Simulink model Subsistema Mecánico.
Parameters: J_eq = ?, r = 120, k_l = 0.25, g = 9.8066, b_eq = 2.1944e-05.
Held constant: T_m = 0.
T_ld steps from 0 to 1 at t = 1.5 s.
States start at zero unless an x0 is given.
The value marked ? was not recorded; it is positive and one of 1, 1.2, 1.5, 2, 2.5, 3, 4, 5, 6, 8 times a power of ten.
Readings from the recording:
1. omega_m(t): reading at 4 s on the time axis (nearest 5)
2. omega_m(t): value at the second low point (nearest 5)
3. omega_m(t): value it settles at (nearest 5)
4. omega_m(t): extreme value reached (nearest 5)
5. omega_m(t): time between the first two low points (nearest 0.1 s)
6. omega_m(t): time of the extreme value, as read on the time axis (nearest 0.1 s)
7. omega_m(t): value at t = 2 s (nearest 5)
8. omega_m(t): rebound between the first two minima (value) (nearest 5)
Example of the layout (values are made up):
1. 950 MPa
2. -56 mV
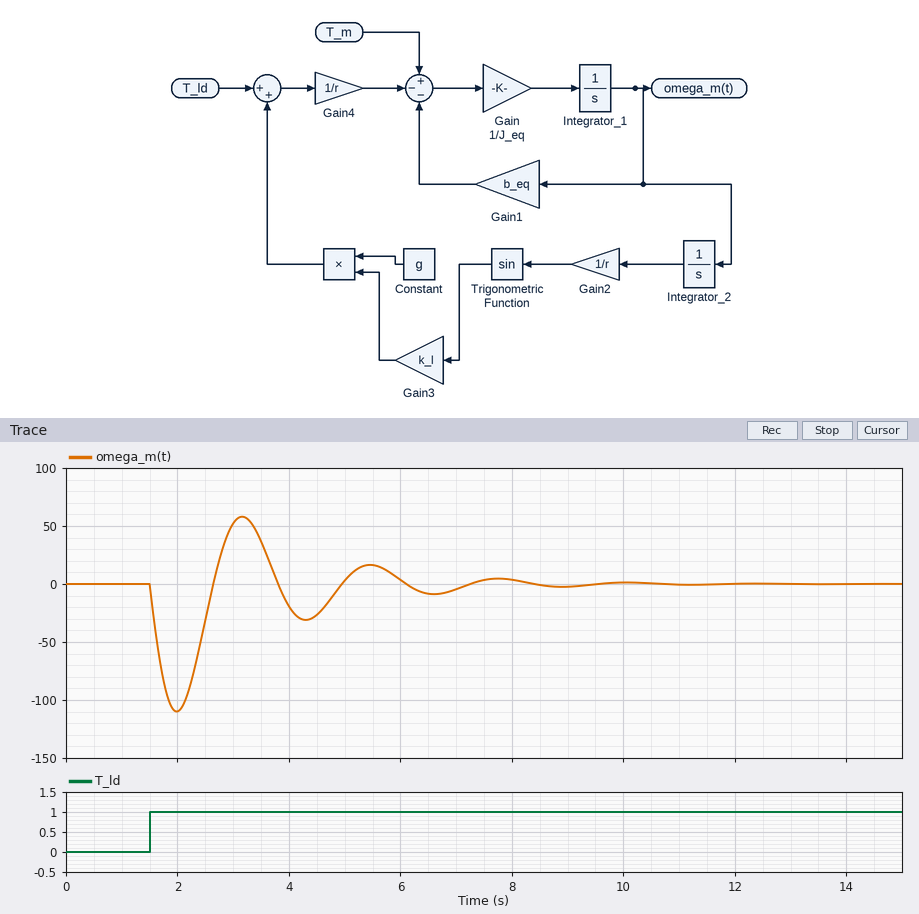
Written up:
1. -20
2. -30
3. 0
4. -110
5. 2.3 s
6. 2.0 s
7. -110
8. 60
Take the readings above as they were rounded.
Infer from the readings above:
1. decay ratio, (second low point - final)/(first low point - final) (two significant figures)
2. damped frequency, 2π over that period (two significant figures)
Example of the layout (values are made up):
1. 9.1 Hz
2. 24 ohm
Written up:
1. 0.27
2. 2.7 rad/s
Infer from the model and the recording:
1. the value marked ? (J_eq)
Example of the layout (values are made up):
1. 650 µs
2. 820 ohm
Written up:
1. 2e-05
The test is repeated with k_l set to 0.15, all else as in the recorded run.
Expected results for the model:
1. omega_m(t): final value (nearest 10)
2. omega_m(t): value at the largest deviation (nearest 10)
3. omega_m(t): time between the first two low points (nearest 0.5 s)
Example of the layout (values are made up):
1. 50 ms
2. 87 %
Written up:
1. 0
2. -130
3. 3.5 s
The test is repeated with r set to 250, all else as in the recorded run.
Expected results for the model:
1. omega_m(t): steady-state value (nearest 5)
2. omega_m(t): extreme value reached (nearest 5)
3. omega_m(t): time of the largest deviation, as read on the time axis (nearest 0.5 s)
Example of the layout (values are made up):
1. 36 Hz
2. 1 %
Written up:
1. 0
2. -85
3. 2.5 s
